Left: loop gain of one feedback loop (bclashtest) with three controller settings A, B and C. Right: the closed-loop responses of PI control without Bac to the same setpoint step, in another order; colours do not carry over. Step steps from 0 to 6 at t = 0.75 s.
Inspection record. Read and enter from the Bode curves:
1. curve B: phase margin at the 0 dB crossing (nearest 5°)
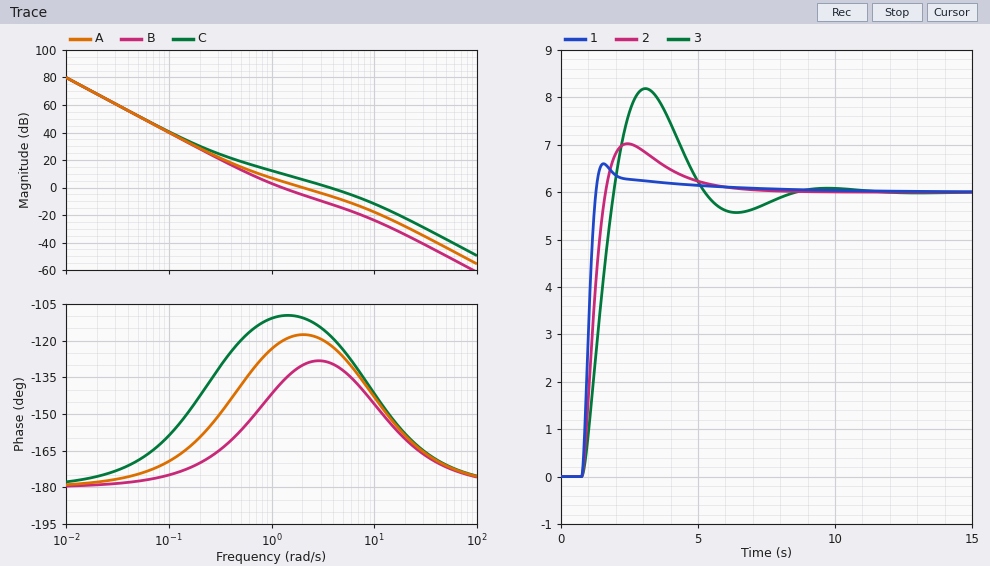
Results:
45°
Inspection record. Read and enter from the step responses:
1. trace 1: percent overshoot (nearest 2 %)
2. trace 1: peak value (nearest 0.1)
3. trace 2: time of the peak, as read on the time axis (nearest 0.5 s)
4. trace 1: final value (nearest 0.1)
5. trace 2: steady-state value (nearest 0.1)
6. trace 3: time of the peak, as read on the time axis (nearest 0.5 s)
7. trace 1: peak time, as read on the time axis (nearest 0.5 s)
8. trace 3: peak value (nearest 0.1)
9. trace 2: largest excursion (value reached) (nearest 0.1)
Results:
10 %
6.6
2.5 s
6.0
6.0
3.0 s
1.5 s
8.2
7.0
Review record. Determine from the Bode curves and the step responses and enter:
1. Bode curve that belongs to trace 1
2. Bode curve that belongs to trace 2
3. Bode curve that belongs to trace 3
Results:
C
A
B
